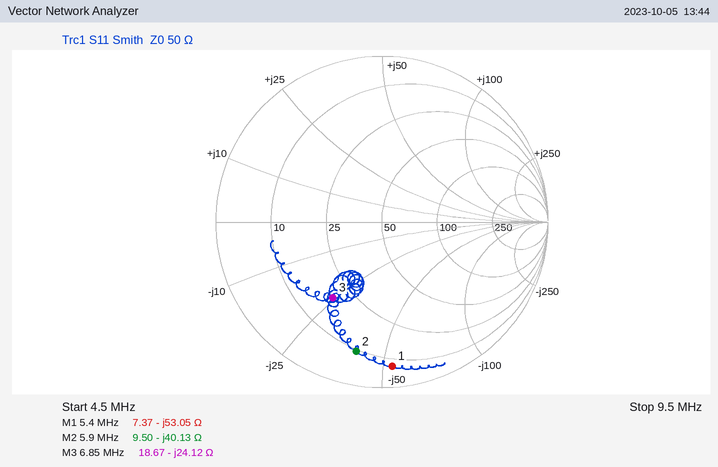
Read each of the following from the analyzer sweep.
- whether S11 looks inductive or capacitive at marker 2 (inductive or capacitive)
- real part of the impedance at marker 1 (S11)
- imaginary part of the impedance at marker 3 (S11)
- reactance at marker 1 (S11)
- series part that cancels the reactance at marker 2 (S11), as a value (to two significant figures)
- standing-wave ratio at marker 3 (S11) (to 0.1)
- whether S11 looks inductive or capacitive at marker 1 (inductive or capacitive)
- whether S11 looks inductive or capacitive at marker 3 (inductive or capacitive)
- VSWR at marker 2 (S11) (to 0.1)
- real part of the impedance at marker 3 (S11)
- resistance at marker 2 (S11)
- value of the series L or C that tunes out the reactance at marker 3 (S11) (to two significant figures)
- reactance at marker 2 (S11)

capacitive
7.37 Ω
-24.12 Ω
-53.05 Ω
1.1 µH
3.4
capacitive
capacitive
8.7
18.67 Ω
9.50 Ω
560 nH
-40.13 Ω
